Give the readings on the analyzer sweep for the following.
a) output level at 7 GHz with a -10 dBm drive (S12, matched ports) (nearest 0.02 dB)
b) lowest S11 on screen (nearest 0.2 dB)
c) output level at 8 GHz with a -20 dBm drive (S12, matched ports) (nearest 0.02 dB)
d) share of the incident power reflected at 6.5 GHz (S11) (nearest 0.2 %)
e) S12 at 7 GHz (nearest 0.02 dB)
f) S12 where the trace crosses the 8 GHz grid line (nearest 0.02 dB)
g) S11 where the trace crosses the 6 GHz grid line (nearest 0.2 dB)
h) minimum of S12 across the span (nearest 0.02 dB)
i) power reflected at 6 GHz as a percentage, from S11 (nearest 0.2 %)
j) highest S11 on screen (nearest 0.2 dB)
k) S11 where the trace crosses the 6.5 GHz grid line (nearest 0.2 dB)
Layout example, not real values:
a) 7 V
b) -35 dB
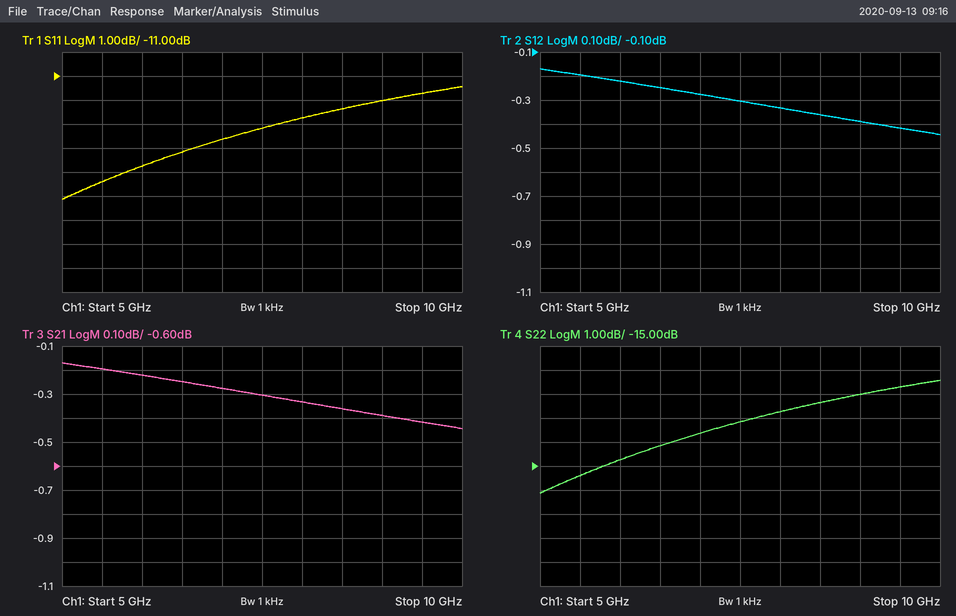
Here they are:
a) -10.28 dBm
b) -16.2 dB
c) -20.34 dBm
d) 3.8 %
e) -0.28 dB
f) -0.34 dB
g) -14.8 dB
h) -0.44 dB
i) 3.4 %
j) -11.4 dB
k) -14.2 dB
